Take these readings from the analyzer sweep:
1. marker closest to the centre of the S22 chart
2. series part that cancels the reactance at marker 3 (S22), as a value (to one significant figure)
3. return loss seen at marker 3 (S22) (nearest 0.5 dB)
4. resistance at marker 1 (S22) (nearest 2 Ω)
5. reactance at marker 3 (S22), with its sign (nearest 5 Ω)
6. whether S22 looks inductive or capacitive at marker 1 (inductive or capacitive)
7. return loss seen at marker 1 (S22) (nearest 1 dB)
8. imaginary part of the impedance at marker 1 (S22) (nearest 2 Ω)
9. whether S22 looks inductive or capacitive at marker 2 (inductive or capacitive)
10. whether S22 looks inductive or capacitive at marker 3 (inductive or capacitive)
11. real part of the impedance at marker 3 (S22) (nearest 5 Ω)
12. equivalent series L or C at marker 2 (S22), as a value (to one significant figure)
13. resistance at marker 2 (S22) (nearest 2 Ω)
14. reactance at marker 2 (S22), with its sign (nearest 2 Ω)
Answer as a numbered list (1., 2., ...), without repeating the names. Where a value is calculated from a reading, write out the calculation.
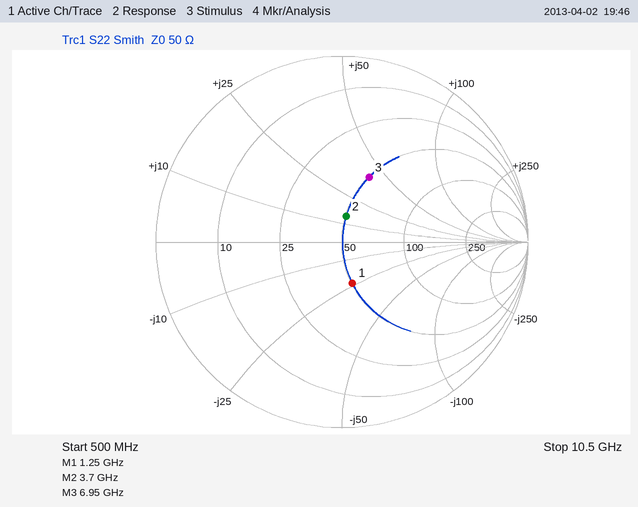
1. marker 2
2. C = 1/(2π × 6.95 GHz × 40 Ω) ≈ 572 fF, so 600 fF to one significant figure
3. 8.5 dB
4. 50 Ω
5. +40 Ω
6. capacitive
7. 13 dB
8. -24 Ω
9. inductive
10. inductive
11. 50 Ω
12. L = 14 Ω/(2π × 3.7 GHz) ≈ 602 pH, so 600 pH to one significant figure
13. 50 Ω
14. +14 Ω
